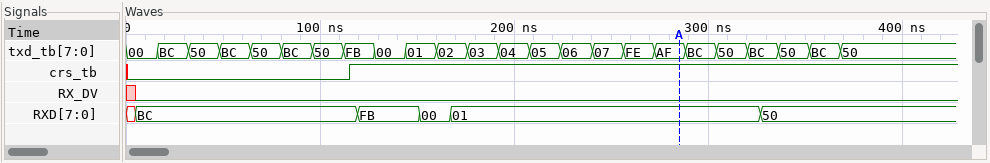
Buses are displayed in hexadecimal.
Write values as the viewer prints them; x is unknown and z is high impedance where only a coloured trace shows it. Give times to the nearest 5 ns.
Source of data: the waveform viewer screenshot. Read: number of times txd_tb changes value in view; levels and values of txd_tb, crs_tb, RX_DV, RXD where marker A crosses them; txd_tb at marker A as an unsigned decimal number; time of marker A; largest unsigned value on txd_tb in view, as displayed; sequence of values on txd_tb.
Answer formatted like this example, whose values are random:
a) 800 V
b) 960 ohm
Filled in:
a) 23
b) txd_tb=AF, crs_tb=1, RX_DV=0, RXD=01
c) 175
d) 285 ns
e) FE
f) 00, BC, 50, BC, 50, BC, 50, FB, 00, 01, 02, 03, 04, 05, 06, 07, FE, AF, BC, 50, BC, 50, BC, 50
